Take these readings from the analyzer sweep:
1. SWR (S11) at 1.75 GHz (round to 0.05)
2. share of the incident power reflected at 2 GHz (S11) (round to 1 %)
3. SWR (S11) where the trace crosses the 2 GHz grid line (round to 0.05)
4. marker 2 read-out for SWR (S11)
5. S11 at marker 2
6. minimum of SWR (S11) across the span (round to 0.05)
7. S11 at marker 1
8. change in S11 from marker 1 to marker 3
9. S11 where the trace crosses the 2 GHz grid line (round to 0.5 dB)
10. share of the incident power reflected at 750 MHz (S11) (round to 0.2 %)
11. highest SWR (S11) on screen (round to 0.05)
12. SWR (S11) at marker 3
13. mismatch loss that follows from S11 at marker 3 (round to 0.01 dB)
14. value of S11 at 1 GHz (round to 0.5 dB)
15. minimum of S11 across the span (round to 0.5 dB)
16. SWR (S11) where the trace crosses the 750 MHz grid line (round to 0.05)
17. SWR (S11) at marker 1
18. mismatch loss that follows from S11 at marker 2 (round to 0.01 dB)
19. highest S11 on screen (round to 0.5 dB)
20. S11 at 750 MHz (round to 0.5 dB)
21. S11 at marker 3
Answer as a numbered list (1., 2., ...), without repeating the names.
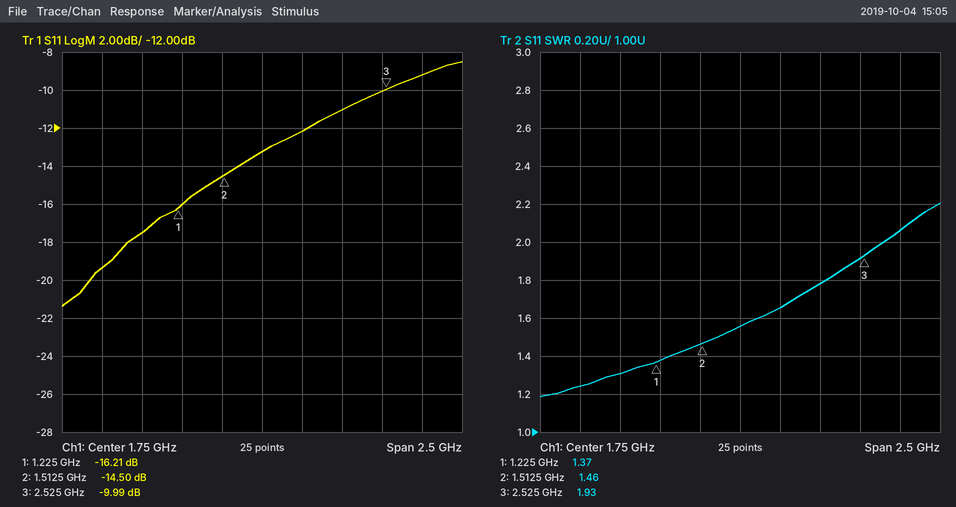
1. 1.55
2. 6 %
3. 1.65
4. 1.46
5. -14.50 dB
6. 1.20
7. -16.21 dB
8. 6.22 dB
9. -12.0 dB
10. 1.2 %
11. 2.20
12. 1.93
13. 0.46 dB
14. -17.5 dB
15. -21.5 dB
16. 1.25
17. 1.37
18. 0.16 dB
19. -8.5 dB
20. -19.5 dB
21. -9.99 dB
